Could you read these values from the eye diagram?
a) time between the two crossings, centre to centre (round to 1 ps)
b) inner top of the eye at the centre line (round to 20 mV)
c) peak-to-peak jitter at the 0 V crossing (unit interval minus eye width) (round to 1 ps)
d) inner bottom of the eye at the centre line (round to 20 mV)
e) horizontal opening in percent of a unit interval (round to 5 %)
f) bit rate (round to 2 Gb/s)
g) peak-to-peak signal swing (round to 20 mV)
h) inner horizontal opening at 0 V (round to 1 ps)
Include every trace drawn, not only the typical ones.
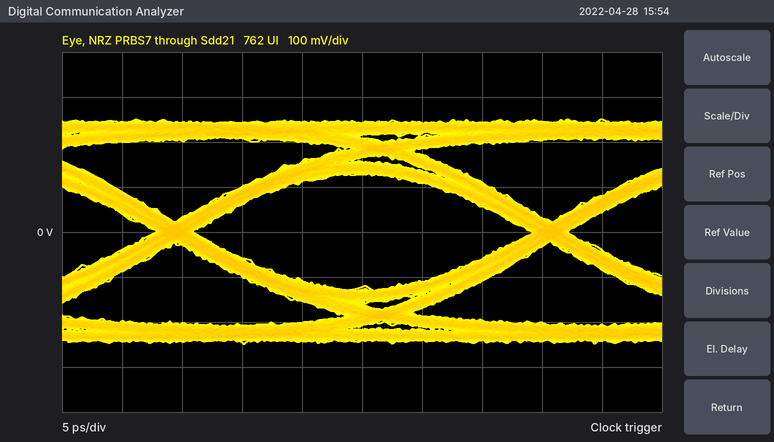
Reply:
31 ps
120 mV
3 ps
-120 mV
90 %
32 Gb/s
500 mV
28 ps
